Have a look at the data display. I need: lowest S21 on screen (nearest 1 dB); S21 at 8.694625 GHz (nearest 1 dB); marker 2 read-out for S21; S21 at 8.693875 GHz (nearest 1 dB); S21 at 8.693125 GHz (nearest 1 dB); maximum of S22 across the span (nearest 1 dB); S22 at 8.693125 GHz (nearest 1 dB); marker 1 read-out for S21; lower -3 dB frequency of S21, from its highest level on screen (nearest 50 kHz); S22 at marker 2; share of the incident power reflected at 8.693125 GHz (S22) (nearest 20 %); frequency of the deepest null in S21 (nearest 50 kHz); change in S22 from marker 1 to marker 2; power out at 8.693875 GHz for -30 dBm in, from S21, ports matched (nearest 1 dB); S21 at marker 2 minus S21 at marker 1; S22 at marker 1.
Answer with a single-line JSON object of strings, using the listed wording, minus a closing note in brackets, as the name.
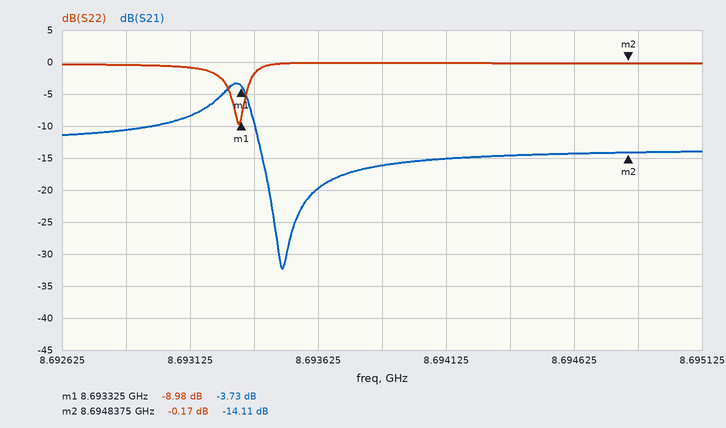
{"lowest S21 on screen": "-32 dB", "S21 at 8.694625 GHz": "-14 dB", "marker 2 read-out for S21": "-14.11 dB", "S21 at 8.693875 GHz": "-16 dB", "S21 at 8.693125 GHz": "-8 dB", "maximum of S22 across the span": "0 dB", "S22 at 8.693125 GHz": "-1 dB", "marker 1 read-out for S21": "-3.73 dB", "lower -3 dB frequency of S21, from its highest level on screen": "8.69320 GHz", "S22 at marker 2": "-0.17 dB", "share of the incident power reflected at 8.693125 GHz (S22)": "80 %", "frequency of the deepest null in S21": "8.69350 GHz", "change in S22 from marker 1 to marker 2": "8.81 dB", "power out at 8.693875 GHz for -30 dBm in, from S21, ports matched": "-46 dBm", "S21 at marker 2 minus S21 at marker 1": "-10.38 dB", "S22 at marker 1": "-8.98 dB"}
